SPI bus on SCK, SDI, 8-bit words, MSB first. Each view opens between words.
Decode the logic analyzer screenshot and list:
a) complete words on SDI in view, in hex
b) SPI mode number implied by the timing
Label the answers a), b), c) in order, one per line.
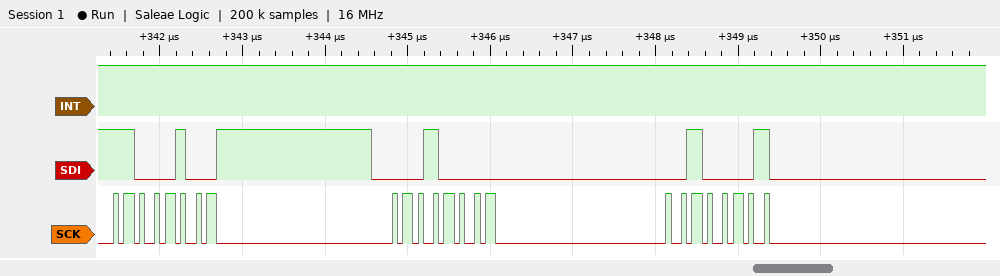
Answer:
a) C4, 10, 21
b) 0
